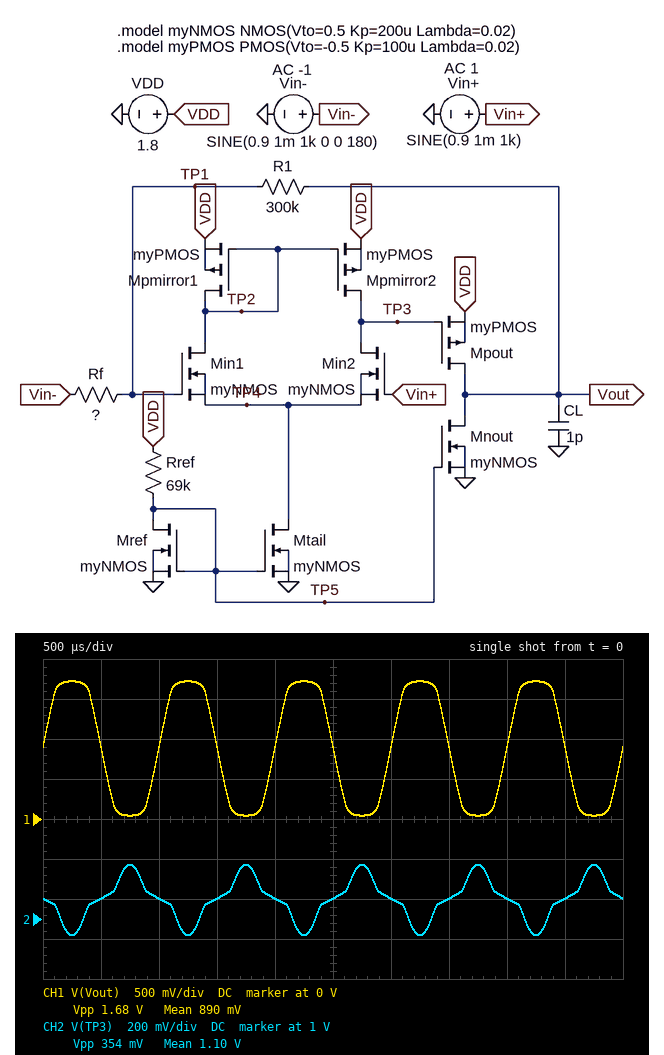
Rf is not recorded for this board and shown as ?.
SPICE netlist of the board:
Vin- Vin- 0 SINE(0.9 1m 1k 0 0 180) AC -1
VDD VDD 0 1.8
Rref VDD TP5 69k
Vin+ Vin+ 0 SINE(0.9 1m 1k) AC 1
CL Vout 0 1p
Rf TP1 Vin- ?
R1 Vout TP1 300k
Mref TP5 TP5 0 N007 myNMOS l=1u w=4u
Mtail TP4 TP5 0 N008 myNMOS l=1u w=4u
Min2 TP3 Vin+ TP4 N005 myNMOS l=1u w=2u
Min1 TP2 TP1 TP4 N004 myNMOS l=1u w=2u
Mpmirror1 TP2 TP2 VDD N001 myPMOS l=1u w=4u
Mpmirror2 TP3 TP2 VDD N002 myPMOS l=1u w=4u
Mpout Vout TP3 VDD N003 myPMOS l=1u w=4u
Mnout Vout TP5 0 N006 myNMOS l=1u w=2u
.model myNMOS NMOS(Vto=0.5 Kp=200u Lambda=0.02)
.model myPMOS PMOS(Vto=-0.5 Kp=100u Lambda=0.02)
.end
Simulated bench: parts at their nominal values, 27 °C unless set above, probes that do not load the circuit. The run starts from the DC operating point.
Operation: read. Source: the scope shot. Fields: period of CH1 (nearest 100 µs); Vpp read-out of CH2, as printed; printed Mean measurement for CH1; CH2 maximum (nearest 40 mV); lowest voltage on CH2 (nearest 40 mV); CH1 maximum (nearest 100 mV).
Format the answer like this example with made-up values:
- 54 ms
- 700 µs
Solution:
- 1.0 ms
- 354 mV
- 890 mV
- 1.28 V
- 920 mV
- 1.7 V
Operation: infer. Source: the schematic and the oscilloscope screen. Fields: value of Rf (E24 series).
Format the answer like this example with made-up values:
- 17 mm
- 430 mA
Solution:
- 470 Ω
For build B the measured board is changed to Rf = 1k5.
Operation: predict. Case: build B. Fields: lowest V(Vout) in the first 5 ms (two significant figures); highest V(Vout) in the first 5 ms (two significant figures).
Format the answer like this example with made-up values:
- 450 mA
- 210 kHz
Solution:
- 510 mV
- 1.3 V
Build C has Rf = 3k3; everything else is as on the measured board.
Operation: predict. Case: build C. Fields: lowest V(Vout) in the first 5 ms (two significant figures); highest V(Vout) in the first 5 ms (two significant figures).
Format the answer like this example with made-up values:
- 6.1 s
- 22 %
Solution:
- 720 mV
- 1.1 V
